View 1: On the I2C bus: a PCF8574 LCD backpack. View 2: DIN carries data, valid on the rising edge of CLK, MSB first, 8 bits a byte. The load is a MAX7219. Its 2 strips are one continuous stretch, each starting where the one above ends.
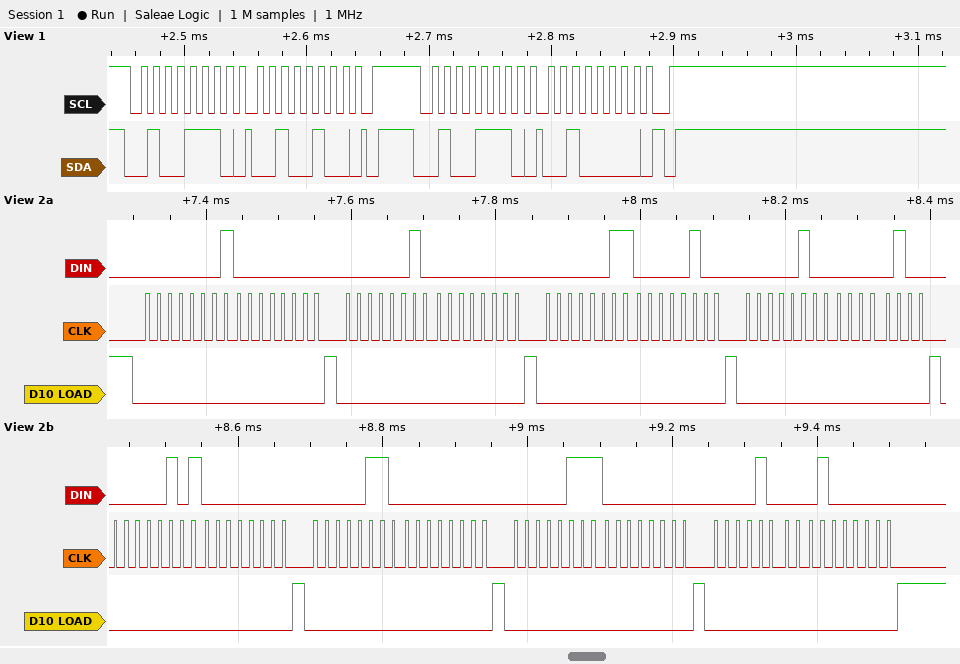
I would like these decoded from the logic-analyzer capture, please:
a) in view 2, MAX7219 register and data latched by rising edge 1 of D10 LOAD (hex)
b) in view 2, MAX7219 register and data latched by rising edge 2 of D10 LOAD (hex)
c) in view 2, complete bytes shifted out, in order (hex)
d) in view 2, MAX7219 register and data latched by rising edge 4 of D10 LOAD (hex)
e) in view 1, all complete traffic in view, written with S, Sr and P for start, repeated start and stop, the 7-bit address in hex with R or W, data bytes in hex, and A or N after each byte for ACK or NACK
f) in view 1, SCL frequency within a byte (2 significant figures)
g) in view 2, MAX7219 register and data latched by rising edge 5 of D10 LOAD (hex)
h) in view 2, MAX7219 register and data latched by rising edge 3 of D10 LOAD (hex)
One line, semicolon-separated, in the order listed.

register 0x1, data 0x00; register 0x2, data 0x00; 01 00 02 00 03 04 04 04 05 00 06 00 07 00 08 40; register 0x4, data 0x04; S 27W A 24 A P S 27W A 20 A P; 100 kHz; register 0x5, data 0x00; register 0x3, data 0x04
